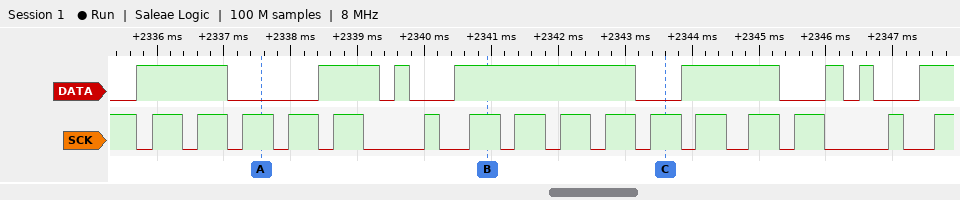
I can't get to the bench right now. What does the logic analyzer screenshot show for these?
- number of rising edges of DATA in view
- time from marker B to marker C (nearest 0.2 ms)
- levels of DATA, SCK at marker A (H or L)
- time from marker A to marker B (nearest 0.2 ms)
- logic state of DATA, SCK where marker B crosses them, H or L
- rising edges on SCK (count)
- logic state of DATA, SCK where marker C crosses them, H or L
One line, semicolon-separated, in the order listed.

8; 2.6 ms; DATA=L, SCK=H; 3.4 ms; DATA=H, SCK=H; 16; DATA=L, SCK=H
